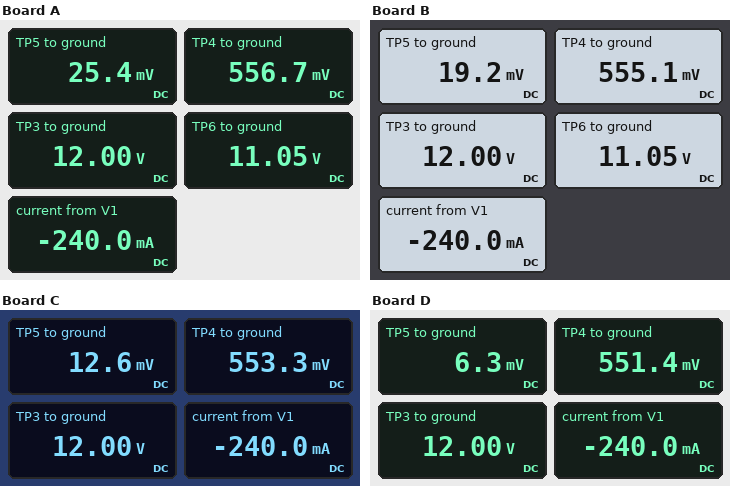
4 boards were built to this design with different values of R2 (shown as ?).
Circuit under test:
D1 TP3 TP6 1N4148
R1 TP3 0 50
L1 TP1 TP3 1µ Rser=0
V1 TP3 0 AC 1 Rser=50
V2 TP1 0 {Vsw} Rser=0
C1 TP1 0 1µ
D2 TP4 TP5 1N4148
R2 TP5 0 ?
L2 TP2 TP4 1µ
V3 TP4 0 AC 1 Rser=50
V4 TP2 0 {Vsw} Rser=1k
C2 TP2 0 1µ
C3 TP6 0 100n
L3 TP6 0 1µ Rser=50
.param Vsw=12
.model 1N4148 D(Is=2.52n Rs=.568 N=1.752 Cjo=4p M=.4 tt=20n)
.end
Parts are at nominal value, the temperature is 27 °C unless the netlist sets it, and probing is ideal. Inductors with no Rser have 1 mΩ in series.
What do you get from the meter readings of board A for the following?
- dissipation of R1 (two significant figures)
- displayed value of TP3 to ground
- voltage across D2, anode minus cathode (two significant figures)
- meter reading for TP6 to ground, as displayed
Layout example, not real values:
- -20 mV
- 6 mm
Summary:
- 2.9 W
- 12.00 V
- 530 mV
- 11.05 V
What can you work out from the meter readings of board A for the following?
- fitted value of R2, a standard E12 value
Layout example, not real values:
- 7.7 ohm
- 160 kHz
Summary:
- 82 Ω
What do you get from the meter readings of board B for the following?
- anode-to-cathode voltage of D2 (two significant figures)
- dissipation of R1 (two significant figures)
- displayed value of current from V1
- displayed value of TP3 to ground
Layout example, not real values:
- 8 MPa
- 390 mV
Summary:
- 540 mV
- 2.9 W
- -240.0 mA
- 12.00 V
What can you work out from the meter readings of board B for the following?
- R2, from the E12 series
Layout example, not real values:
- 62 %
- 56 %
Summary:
- 56 Ω
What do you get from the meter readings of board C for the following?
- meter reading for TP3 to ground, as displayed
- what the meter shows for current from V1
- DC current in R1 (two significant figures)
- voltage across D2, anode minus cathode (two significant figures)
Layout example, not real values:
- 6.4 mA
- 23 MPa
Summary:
- 12.00 V
- -240.0 mA
- 240 mA
- 540 mV
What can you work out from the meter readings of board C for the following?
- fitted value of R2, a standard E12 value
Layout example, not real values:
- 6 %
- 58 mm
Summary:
- 33 Ω
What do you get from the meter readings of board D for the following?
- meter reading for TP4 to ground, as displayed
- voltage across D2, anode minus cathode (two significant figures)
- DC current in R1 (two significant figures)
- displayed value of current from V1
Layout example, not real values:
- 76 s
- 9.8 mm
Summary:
- 551.4 mV
- 550 mV
- 240 mA
- -240.0 mA
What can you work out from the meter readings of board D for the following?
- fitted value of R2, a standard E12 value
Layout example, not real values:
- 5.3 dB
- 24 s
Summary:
- 15 Ω
